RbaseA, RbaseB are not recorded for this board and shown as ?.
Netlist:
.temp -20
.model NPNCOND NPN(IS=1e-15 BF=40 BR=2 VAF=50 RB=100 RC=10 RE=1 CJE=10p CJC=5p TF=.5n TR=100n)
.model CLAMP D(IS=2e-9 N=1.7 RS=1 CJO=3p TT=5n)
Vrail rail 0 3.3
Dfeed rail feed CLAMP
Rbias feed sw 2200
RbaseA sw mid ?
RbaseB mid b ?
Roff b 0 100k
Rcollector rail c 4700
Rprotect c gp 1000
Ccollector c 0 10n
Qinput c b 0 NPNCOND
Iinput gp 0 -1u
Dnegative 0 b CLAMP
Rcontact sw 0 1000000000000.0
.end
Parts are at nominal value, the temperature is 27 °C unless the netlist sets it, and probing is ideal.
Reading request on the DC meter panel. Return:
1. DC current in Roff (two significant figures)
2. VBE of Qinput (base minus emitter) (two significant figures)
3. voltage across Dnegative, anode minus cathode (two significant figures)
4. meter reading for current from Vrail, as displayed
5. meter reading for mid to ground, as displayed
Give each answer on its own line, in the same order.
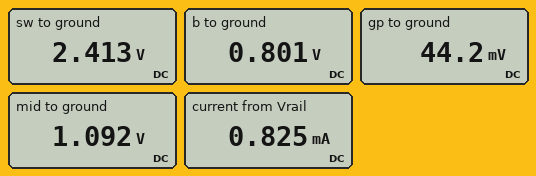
8.0 µA
800 mV
-800 mV
0.825 mA
1.092 V
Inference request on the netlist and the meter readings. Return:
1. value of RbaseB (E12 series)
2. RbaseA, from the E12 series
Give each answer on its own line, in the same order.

2.2 kΩ
10 kΩ
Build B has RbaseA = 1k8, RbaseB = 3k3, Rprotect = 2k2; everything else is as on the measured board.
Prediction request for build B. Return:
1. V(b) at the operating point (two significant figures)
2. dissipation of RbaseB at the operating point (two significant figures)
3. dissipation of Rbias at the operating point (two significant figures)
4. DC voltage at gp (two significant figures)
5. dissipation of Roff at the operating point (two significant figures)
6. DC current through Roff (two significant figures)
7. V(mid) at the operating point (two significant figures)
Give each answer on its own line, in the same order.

820 mV
210 µW
140 µW
35 mV
6.7 µW
8.2 µA
1.7 V
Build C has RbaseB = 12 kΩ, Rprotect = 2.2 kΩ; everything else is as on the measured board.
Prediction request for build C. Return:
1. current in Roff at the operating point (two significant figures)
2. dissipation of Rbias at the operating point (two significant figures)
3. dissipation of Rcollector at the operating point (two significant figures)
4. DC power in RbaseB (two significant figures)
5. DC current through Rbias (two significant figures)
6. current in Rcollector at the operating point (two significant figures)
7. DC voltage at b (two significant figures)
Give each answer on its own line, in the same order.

7.9 µA
14 µW
2.2 mW
76 µW
80 µA
690 µA
790 mV
